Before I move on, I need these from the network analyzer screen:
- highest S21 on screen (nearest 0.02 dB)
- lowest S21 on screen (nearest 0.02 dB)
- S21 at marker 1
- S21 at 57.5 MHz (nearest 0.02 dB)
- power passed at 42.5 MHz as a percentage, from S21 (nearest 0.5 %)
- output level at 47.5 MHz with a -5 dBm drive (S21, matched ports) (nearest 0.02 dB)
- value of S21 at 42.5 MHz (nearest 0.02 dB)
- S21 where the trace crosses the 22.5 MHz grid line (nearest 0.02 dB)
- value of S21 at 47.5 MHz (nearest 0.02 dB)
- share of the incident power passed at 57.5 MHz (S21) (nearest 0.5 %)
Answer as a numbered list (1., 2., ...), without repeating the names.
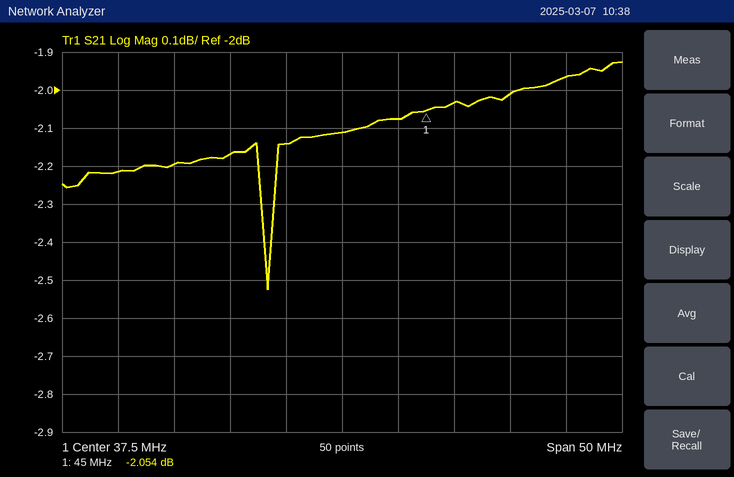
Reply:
1. -1.92 dB
2. -2.52 dB
3. -2.054 dB
4. -1.96 dB
5. 62.0 %
6. -7.04 dBm
7. -2.08 dB
8. -2.20 dB
9. -2.04 dB
10. 63.5 %
